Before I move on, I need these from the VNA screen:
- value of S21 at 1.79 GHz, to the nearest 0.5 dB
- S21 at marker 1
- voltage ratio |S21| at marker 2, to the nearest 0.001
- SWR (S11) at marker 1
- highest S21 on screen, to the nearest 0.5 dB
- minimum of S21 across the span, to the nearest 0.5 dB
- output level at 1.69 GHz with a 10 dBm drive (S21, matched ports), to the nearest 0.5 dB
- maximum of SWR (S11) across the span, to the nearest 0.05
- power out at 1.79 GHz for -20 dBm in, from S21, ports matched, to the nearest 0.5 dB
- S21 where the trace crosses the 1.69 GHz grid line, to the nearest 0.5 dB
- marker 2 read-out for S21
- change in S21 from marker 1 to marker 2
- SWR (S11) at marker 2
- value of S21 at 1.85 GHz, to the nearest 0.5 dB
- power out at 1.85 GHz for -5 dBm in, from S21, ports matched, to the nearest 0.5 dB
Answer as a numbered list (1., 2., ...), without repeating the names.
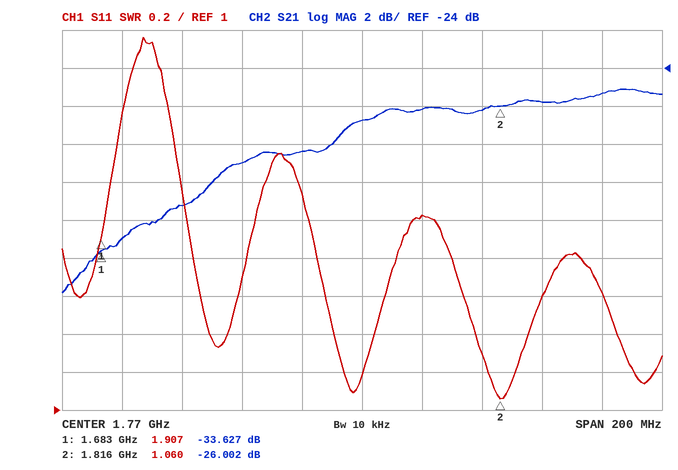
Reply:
1. -26.0 dB
2. -33.627 dB
3. 0.050
4. 1.907
5. -25.0 dB
6. -36.0 dB
7. -23.0 dBm
8. 2.95
9. -46.0 dBm
10. -33.0 dB
11. -26.002 dB
12. 7.625 dB
13. 1.060
14. -25.5 dB
15. -30.5 dBm
